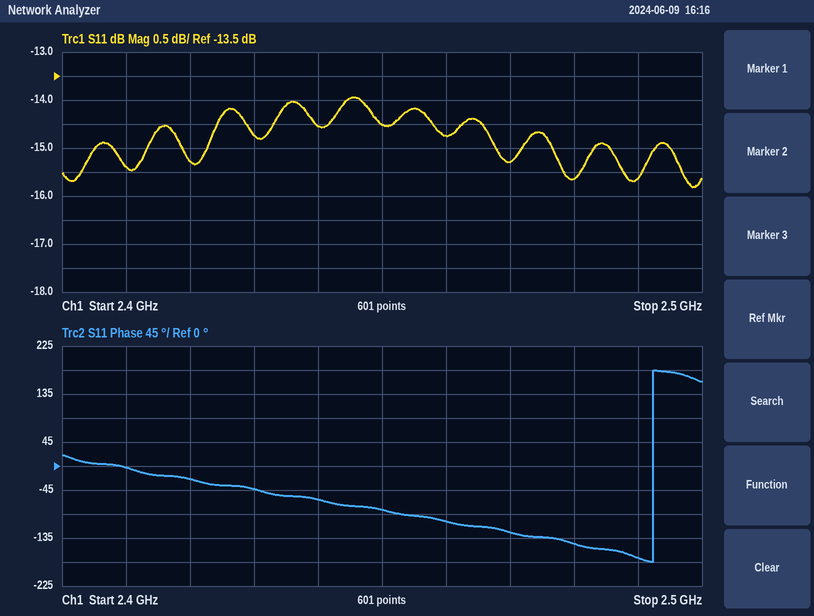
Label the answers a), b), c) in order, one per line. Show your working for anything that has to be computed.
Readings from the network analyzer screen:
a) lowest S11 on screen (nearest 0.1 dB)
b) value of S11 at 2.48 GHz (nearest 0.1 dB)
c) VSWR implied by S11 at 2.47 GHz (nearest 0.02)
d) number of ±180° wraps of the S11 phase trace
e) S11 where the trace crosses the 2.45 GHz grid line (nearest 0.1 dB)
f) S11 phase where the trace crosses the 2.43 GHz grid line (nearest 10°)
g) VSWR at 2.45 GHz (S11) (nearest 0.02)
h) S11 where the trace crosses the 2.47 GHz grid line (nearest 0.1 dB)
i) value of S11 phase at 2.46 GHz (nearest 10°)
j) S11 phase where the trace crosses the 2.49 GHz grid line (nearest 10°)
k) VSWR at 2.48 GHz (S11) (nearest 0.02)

a) -15.8 dB
b) -15.6 dB
c) |Γ| = 10^(-15.3/20) = 0.1718; VSWR = (1 + 0.1718)/(1 − 0.1718) ≈ 1.41, so 1.42 to the nearest 0.02
d) 1
e) -14.5 dB
f) -40°
g) |Γ| = 10^(-14.5/20) = 0.1884; VSWR = (1 + 0.1884)/(1 − 0.1884) ≈ 1.46
h) -15.3 dB
i) -100°
j) -170°
k) |Γ| = 10^(-15.6/20) = 0.1660; VSWR = (1 + 0.1660)/(1 − 0.1660) ≈ 1.40
